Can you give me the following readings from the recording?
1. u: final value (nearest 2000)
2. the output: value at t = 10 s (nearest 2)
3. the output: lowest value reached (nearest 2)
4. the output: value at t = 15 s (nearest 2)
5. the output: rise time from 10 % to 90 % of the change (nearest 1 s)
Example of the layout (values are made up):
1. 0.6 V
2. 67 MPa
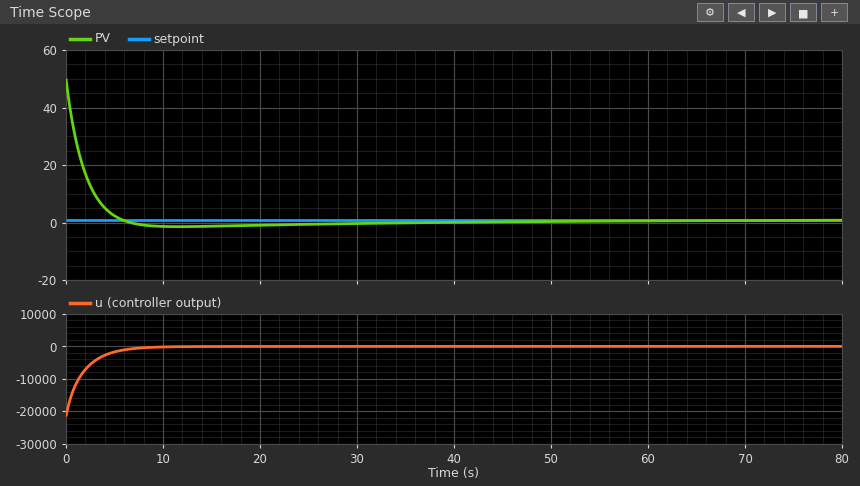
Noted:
1. 0
2. -2
3. -2
4. -2
5. 4 s
